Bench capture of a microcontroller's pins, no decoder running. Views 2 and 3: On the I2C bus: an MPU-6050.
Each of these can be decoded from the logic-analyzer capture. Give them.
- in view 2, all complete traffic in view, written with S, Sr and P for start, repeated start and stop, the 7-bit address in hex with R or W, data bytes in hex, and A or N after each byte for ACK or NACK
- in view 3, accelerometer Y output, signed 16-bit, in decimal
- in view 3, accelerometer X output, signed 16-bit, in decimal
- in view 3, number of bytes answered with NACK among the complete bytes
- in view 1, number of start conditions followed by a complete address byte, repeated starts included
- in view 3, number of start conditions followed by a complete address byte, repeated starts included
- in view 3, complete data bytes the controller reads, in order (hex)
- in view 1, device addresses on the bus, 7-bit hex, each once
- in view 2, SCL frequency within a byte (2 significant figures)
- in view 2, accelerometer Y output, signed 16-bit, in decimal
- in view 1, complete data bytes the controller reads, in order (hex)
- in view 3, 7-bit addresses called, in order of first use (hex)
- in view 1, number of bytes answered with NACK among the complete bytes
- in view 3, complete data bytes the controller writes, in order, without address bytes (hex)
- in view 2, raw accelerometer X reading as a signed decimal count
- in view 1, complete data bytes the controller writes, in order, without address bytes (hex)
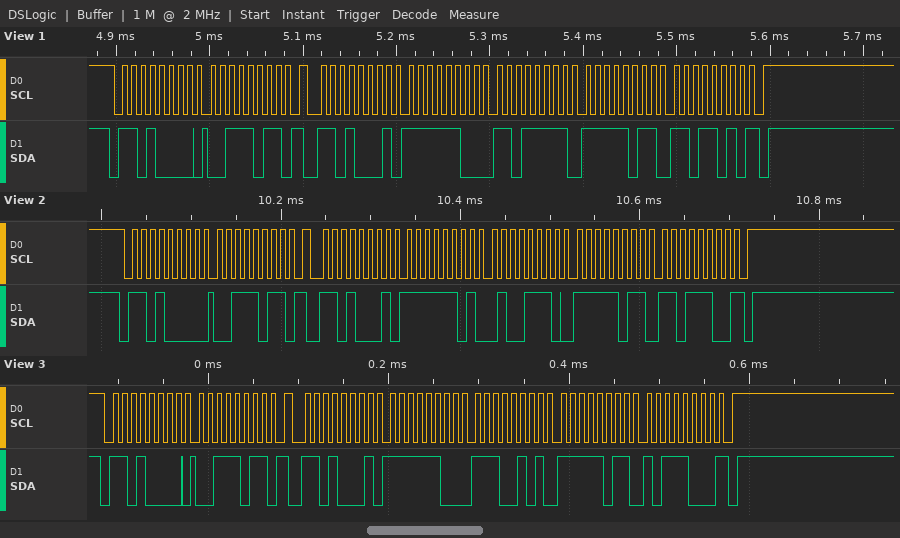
S 68W A 3B A Sr 68R A FD A 4E A FB A DC N P
-1096
-795
1
2
2
FC E5 FB B8
0x68
100 kHz
-1060
FC DF FB DA
0x68
1
3B
-690
3B
